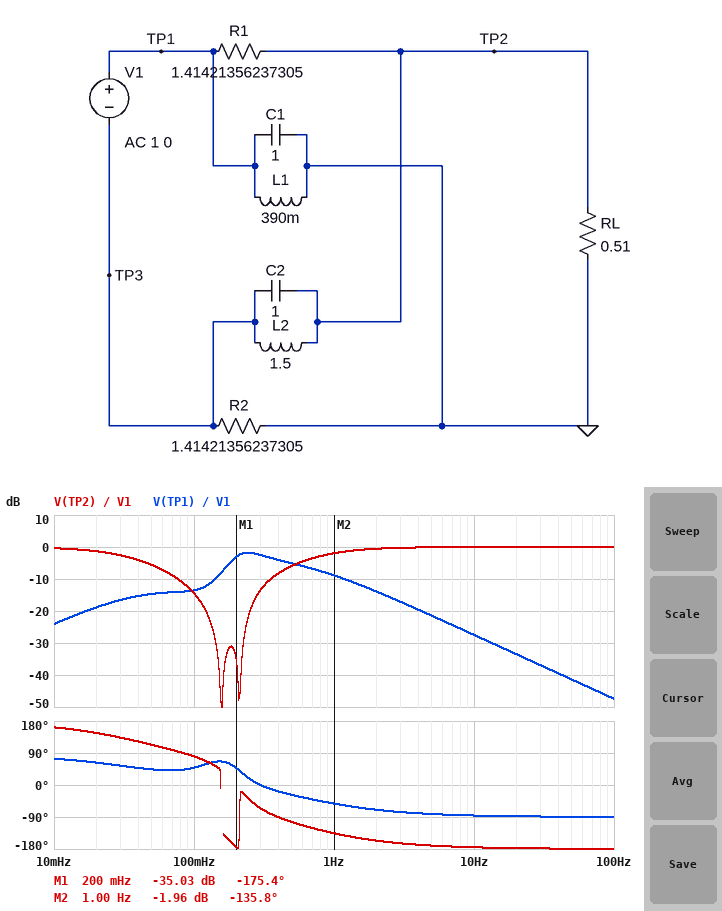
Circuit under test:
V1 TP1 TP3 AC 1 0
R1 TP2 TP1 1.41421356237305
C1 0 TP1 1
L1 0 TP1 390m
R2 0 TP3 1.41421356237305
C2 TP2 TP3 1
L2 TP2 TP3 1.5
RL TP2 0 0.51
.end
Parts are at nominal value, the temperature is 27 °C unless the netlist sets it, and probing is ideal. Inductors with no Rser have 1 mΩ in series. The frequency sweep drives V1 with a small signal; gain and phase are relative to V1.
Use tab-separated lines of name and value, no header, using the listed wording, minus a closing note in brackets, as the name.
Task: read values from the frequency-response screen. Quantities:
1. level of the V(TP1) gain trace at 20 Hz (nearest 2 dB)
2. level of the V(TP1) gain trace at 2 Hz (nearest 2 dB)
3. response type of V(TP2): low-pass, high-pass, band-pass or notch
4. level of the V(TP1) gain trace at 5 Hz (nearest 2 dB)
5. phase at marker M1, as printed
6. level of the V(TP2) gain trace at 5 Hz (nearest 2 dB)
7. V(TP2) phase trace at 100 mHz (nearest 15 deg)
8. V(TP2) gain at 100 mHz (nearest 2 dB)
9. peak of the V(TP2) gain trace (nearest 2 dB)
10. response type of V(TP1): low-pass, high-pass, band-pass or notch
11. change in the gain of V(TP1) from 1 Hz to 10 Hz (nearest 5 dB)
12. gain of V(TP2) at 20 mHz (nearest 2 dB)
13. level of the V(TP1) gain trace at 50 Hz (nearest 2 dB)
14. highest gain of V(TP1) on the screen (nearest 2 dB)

level of the V(TP1) gain trace at 20 Hz	-34 dB
level of the V(TP1) gain trace at 2 Hz	-14 dB
response type of V(TP2): low-pass, high-pass, band-pass or notch	notch
level of the V(TP1) gain trace at 5 Hz	-22 dB
phase at marker M1, as printed	-175.4 deg
level of the V(TP2) gain trace at 5 Hz	0 dB
V(TP2) phase trace at 100 mHz	75 deg
V(TP2) gain at 100 mHz	-14 dB
peak of the V(TP2) gain trace	0 dB
response type of V(TP1): low-pass, high-pass, band-pass or notch	band-pass
change in the gain of V(TP1) from 1 Hz to 10 Hz	-20 dB
gain of V(TP2) at 20 mHz	-2 dB
level of the V(TP1) gain trace at 50 Hz	-42 dB
highest gain of V(TP1) on the screen	-2 dB
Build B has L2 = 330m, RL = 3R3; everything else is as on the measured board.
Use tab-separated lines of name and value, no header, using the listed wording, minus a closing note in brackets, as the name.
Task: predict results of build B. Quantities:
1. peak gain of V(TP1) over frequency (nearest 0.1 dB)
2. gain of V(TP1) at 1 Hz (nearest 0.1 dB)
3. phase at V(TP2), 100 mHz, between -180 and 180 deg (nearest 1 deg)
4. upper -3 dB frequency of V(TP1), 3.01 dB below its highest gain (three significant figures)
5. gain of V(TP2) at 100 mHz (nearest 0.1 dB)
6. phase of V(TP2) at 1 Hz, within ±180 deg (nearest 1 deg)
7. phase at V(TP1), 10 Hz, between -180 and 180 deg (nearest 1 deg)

peak gain of V(TP1) over frequency	-1.9 dB
gain of V(TP1) at 1 Hz	-15.5 dB
phase at V(TP2), 100 mHz, between -180 and 180 deg	150 deg
upper -3 dB frequency of V(TP1), 3.01 dB below its highest gain	359 mHz
gain of V(TP2) at 100 mHz	-0.4 dB
phase of V(TP2) at 1 Hz, within ±180 deg	-160 deg
phase at V(TP1), 10 Hz, between -180 and 180 deg	-89 deg
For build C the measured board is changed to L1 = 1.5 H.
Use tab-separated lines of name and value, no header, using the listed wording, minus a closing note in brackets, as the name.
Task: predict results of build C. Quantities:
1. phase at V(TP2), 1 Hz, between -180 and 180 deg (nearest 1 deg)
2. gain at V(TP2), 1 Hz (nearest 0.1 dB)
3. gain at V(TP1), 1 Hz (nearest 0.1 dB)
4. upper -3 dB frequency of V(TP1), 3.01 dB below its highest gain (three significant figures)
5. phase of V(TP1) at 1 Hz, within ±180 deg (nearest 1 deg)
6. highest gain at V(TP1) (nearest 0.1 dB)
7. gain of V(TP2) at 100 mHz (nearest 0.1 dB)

phase at V(TP2), 1 Hz, between -180 and 180 deg	-137 deg
gain at V(TP2), 1 Hz	-1.9 dB
gain at V(TP1), 1 Hz	-9.2 dB
upper -3 dB frequency of V(TP1), 3.01 dB below its highest gain	759 mHz
phase of V(TP1) at 1 Hz, within ±180 deg	-53 deg
highest gain at V(TP1)	-4.8 dB
gain of V(TP2) at 100 mHz	-15.0 dB
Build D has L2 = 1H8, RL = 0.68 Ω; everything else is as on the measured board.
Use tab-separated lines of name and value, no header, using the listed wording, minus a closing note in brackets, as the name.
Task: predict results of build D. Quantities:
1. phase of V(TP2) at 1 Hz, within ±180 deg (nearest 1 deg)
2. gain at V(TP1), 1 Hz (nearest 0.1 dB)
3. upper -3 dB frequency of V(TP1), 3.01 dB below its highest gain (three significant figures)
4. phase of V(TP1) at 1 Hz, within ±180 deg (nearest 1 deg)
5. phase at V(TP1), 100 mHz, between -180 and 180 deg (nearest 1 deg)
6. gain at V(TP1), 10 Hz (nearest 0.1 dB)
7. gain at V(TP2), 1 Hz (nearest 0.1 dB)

phase of V(TP2) at 1 Hz, within ±180 deg	-142 deg
gain at V(TP1), 1 Hz	-10.0 dB
upper -3 dB frequency of V(TP1), 3.01 dB below its highest gain	437 mHz
phase of V(TP1) at 1 Hz, within ±180 deg	-59 deg
phase at V(TP1), 100 mHz, between -180 and 180 deg	58 deg
gain at V(TP1), 10 Hz	-29.2 dB
gain at V(TP2), 1 Hz	-1.3 dB
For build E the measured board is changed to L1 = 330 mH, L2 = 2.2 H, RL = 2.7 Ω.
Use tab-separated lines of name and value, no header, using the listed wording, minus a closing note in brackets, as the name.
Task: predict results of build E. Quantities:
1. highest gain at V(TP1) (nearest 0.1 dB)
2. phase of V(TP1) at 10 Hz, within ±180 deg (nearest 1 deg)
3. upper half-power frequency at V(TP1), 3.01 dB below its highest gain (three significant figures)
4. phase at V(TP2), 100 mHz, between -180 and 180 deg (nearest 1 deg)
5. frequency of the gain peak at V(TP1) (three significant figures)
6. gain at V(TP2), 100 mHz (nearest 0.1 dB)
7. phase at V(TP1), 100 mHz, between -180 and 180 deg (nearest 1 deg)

highest gain at V(TP1)	-0.6 dB
phase of V(TP1) at 10 Hz, within ±180 deg	-89 deg
upper half-power frequency at V(TP1), 3.01 dB below its highest gain	376 mHz
phase at V(TP2), 100 mHz, between -180 and 180 deg	82 deg
frequency of the gain peak at V(TP1)	276 mHz
gain at V(TP2), 100 mHz	-14.3 dB
phase at V(TP1), 100 mHz, between -180 and 180 deg	74 deg
